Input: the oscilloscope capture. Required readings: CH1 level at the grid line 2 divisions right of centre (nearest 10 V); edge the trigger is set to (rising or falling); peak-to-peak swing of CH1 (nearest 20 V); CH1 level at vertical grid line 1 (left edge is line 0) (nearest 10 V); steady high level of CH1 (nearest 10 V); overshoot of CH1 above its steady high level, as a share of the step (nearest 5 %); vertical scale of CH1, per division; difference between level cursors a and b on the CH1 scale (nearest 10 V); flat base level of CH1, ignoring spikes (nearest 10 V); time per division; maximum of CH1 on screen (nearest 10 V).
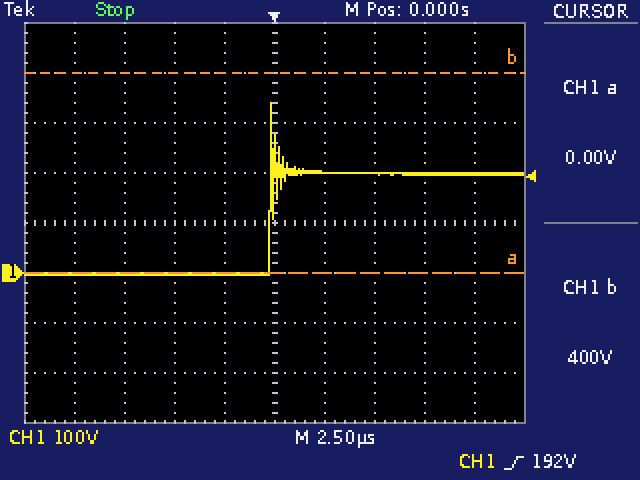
200 V
rising
340 V
0 V
200 V
70 %
100 V
400 V
0 V
2.5 µs
340 V
